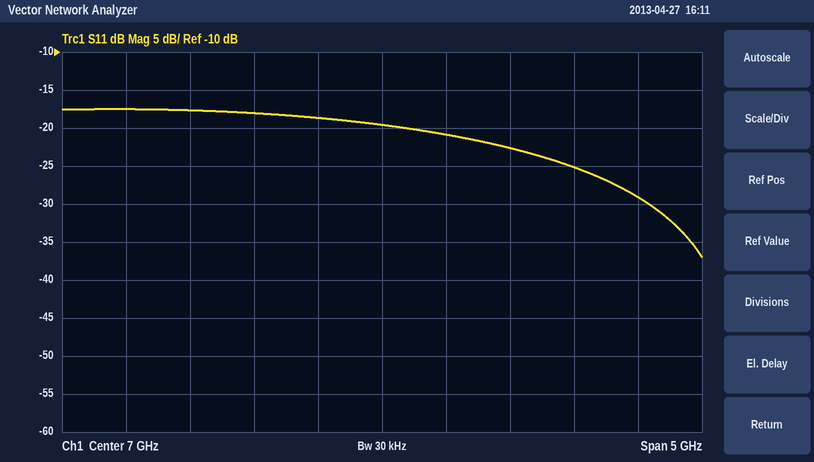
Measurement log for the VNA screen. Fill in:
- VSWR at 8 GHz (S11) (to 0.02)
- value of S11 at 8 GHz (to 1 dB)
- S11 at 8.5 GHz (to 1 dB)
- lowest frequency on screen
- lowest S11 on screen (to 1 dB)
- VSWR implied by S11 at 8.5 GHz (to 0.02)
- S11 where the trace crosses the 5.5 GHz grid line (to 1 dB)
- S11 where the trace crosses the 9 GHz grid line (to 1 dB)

1.16
-23 dB
-25 dB
4.5 GHz
-37 dB
1.12
-18 dB
-29 dB
